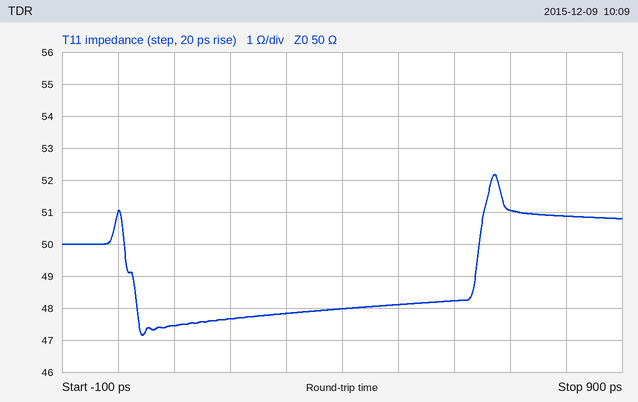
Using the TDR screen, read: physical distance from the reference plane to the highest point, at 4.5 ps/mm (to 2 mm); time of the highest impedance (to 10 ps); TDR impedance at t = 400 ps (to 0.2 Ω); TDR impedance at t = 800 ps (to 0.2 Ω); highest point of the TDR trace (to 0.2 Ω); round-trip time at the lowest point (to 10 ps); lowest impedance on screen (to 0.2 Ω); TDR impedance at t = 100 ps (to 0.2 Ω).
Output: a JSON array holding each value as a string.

["74 mm", "670 ps", "48.0 Ω", "50.8 Ω", "52.2 Ω", "40 ps", "47.2 Ω", "47.4 Ω"]
